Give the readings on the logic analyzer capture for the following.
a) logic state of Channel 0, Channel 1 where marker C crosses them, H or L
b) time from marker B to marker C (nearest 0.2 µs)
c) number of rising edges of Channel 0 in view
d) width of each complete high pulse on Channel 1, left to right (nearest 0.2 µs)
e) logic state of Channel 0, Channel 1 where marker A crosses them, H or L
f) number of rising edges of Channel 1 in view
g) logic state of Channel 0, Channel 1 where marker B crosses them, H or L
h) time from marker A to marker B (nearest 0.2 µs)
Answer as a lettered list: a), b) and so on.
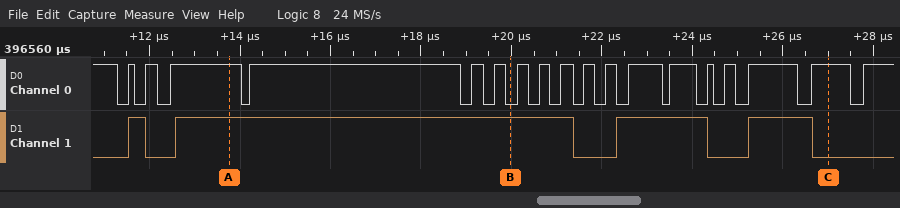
a) Channel 0=H, Channel 1=L
b) 7 µs
c) 18
d) 0.4 µs, 8.8 µs, 2 µs, 1.4 µs
e) Channel 0=H, Channel 1=H
f) 4
g) Channel 0=L, Channel 1=H
h) 6.2 µs
